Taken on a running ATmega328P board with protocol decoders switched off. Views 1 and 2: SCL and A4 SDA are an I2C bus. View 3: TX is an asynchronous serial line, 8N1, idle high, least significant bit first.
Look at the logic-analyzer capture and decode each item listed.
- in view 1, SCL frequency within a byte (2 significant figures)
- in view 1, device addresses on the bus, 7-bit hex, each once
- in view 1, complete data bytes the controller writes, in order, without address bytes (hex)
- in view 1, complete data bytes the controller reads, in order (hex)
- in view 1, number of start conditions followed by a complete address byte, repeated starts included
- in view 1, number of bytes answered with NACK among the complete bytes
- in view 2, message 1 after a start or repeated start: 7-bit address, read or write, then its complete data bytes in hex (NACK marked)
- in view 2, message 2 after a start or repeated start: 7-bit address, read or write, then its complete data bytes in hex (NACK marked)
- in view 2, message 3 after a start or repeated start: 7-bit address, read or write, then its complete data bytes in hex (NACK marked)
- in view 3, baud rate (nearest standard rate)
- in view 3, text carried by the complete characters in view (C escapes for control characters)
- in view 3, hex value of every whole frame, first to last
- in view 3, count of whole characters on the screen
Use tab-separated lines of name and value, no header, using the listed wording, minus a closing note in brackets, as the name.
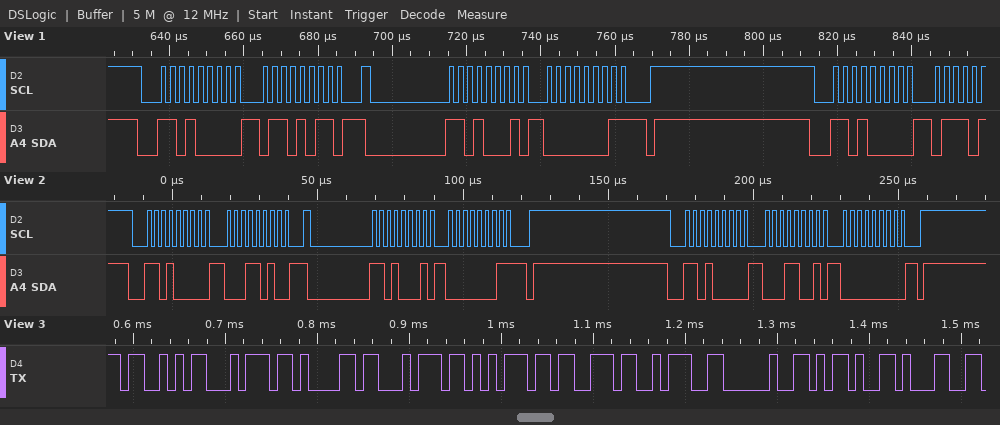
in view 1, SCL frequency within a byte	400 kHz
in view 1, device addresses on the bus, 7-bit hex, each once	0x68
in view 1, complete data bytes the controller writes, in order, without address bytes	6B
in view 1, complete data bytes the controller reads, in order	01
in view 1, number of start conditions followed by a complete address byte, repeated starts included	3
in view 1, number of bytes answered with NACK among the complete bytes	1
in view 2, message 1 after a start or repeated start: 7-bit address, read or write, then its complete data bytes in hex	0x68 write: 1A
in view 2, message 2 after a start or repeated start: 7-bit address, read or write, then its complete data bytes in hex	0x68 read: 01 NACK
in view 2, message 3 after a start or repeated start: 7-bit address, read or write, then its complete data bytes in hex	0x68 write: 19 00
in view 3, baud rate	115200 baud
in view 3, text carried by the complete characters in view	"Status: -1"
in view 3, hex value of every whole frame, first to last	53 74 61 74 75 73 3A 20 2D 31
in view 3, count of whole characters on the screen	10
